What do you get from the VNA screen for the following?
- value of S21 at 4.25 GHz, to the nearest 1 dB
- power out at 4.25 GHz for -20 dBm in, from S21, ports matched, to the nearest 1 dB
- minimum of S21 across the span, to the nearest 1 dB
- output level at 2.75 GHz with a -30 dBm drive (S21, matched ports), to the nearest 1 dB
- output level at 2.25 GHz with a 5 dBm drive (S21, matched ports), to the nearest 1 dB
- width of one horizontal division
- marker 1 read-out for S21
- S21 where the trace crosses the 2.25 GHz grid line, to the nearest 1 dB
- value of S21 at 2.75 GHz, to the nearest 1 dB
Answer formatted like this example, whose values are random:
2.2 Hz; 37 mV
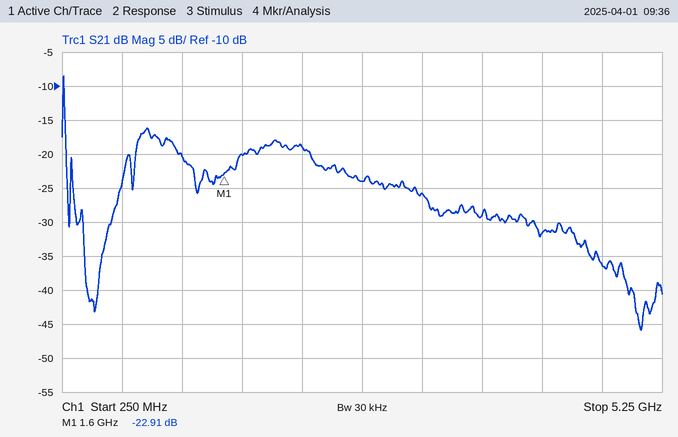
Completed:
-32 dB; -52 dBm; -46 dB; -54 dBm; -14 dBm; 500 MHz; -22.91 dB; -19 dB; -24 dB
